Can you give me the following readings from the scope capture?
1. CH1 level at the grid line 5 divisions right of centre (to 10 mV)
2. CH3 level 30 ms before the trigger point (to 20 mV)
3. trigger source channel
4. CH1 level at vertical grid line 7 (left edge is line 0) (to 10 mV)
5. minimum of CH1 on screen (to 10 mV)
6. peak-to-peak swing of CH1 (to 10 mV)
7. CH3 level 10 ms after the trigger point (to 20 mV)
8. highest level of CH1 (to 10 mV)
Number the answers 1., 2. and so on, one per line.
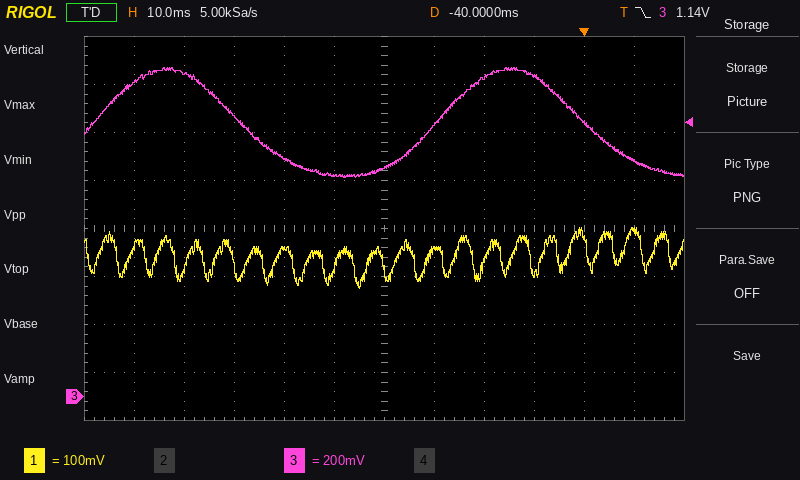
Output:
1. 340 mV
2. 1.14 V
3. CH3
4. 300 mV
5. 220 mV
6. 130 mV
7. 980 mV
8. 350 mV
